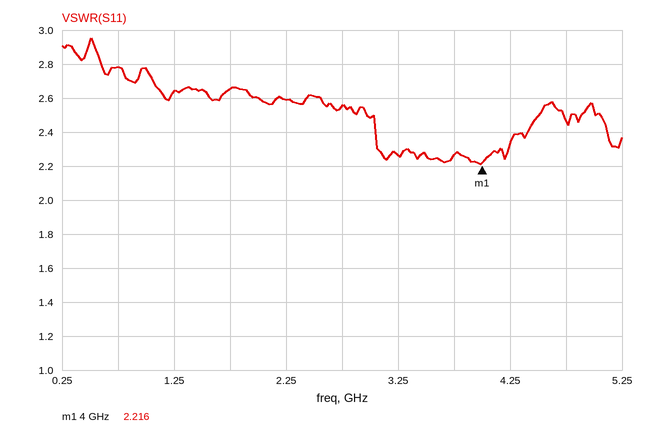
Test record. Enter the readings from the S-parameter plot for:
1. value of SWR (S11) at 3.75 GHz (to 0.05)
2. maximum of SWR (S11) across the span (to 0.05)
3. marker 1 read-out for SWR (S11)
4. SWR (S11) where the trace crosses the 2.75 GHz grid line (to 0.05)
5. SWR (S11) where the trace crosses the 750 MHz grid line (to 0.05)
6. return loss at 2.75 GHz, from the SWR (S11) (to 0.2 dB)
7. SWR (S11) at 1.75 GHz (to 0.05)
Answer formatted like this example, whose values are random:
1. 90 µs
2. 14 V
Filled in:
1. 2.25
2. 2.95
3. 2.216
4. 2.55
5. 2.80
6. 7.2 dB
7. 2.65
